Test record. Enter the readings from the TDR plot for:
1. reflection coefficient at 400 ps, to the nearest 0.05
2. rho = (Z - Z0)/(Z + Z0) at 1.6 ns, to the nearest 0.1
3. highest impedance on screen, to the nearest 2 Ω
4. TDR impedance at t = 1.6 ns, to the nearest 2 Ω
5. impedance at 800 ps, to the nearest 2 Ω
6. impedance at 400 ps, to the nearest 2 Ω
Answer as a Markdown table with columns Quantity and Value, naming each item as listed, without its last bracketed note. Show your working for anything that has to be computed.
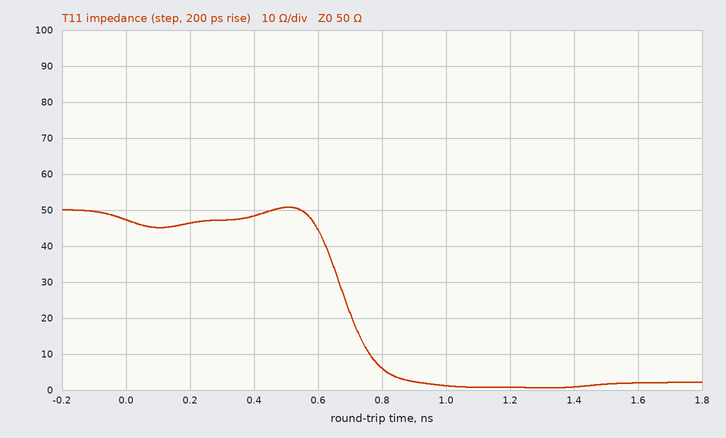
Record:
| Quantity | Value |
|---|---|
| reflection coefficient at 400 ps, to the nearest 0.05 | (48 − 50)/(48 + 50) ≈ 0.00 |
| rho = (Z - Z0)/(Z + Z0) at 1.6 ns, to the nearest 0.1 | (2 − 50)/(2 + 50) ≈ -0.9 |
| highest impedance on screen, to the nearest 2 Ω | 50 Ω |
| TDR impedance at t = 1.6 ns, to the nearest 2 Ω | 2 Ω |
| impedance at 800 ps, to the nearest 2 Ω | 6 Ω |
| impedance at 400 ps, to the nearest 2 Ω | 48 Ω |
